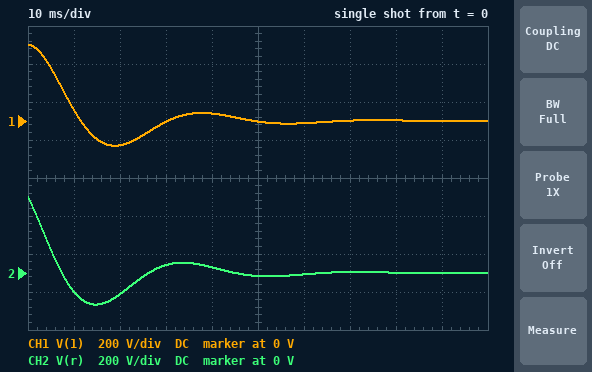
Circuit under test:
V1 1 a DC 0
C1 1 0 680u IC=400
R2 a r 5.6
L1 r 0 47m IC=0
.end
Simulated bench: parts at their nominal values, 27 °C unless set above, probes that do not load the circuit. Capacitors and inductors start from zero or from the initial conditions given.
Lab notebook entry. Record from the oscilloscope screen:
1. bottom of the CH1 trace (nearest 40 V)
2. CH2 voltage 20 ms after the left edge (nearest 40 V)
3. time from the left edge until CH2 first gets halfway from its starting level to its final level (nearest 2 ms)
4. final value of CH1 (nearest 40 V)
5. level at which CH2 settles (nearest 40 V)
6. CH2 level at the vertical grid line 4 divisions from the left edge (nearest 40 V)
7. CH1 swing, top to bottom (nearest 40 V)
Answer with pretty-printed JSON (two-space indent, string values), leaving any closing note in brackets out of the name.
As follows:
{
  "bottom of the CH1 trace": "-120 V",
  "CH2 voltage 20 ms after the left edge": "-120 V",
  "time from the left edge until CH2 first gets halfway from its starting level to its final level": "4 ms",
  "final value of CH1": "0 V",
  "level at which CH2 settles": "0 V",
  "CH2 level at the vertical grid line 4 divisions from the left edge": "40 V",
  "CH1 swing, top to bottom": "520 V"
}
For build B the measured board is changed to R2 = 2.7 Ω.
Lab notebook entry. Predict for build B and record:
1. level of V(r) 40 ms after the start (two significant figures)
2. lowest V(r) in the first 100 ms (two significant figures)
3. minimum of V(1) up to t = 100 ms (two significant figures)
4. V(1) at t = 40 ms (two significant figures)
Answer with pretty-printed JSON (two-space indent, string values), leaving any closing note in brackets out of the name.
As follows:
{
  "level of V(r) 40 ms after the start": "84 V",
  "lowest V(r) in the first 100 ms": "-250 V",
  "minimum of V(1) up to t = 100 ms": "-240 V",
  "V(1) at t = 40 ms": "110 V"
}
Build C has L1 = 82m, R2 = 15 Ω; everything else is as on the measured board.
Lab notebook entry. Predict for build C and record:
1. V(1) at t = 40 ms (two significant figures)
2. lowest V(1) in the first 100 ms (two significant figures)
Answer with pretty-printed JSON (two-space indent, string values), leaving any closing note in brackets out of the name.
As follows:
{
  "V(1) at t = 40 ms": "-14 V",
  "lowest V(1) in the first 100 ms": "-21 V"
}
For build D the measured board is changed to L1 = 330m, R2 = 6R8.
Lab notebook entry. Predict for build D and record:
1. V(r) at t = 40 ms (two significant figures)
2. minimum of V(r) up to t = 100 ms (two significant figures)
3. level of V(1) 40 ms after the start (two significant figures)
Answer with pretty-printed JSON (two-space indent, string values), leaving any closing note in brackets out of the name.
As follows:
{
  "V(r) at t = 40 ms": "-250 V",
  "minimum of V(r) up to t = 100 ms": "-260 V",
  "level of V(1) 40 ms after the start": "-210 V"
}
